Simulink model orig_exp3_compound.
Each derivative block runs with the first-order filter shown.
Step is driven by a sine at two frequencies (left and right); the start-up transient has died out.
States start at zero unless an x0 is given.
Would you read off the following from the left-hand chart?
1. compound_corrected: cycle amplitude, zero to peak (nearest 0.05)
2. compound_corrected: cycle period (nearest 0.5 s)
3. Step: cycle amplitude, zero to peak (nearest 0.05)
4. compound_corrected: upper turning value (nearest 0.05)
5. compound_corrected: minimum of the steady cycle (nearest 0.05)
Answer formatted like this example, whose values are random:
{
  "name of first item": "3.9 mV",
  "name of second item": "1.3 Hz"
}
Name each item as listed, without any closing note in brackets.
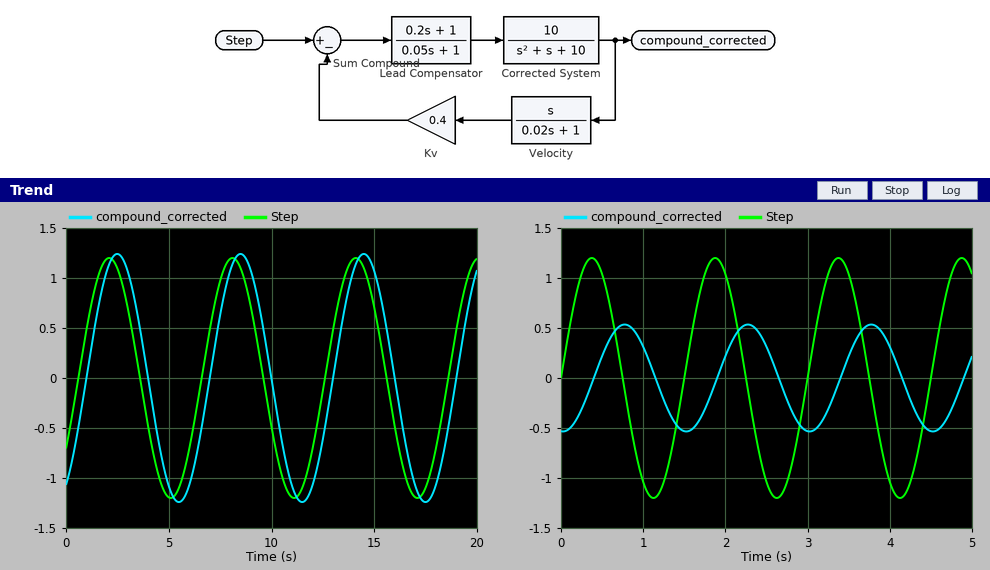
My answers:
{
  "compound_corrected: cycle amplitude, zero to peak": "1.25",
  "compound_corrected: cycle period": "6.0 s",
  "Step: cycle amplitude, zero to peak": "1.20",
  "compound_corrected: upper turning value": "1.25",
  "compound_corrected: minimum of the steady cycle": "-1.25"
}
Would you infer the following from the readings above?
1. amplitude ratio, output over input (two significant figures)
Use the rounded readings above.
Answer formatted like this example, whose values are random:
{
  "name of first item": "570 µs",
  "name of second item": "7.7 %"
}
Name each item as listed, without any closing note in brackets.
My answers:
{
  "amplitude ratio, output over input": "1.0"
}
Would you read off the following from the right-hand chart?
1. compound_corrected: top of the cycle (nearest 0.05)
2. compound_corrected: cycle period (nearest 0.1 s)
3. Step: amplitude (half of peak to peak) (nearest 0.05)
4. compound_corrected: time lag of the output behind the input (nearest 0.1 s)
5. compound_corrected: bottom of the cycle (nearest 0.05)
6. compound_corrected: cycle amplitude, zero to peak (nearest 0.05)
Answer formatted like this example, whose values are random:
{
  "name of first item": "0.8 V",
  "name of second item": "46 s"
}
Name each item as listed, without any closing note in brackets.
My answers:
{
  "compound_corrected: top of the cycle": "0.55",
  "compound_corrected: cycle period": "1.5 s",
  "Step: amplitude (half of peak to peak)": "1.20",
  "compound_corrected: time lag of the output behind the input": "0.4 s",
  "compound_corrected: bottom of the cycle": "-0.55",
  "compound_corrected: cycle amplitude, zero to peak": "0.55"
}
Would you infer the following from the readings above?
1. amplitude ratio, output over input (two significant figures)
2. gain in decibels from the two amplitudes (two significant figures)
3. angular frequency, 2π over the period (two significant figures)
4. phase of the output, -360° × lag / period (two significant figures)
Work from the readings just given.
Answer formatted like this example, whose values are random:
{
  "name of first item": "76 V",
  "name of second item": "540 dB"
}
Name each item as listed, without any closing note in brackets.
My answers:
{
  "amplitude ratio, output over input": "0.46",
  "gain in decibels from the two amplitudes": "-6.8 dB",
  "angular frequency, 2π over the period": "4.2 rad/s",
  "phase of the output, -360° × lag / period": "-96°"
}
